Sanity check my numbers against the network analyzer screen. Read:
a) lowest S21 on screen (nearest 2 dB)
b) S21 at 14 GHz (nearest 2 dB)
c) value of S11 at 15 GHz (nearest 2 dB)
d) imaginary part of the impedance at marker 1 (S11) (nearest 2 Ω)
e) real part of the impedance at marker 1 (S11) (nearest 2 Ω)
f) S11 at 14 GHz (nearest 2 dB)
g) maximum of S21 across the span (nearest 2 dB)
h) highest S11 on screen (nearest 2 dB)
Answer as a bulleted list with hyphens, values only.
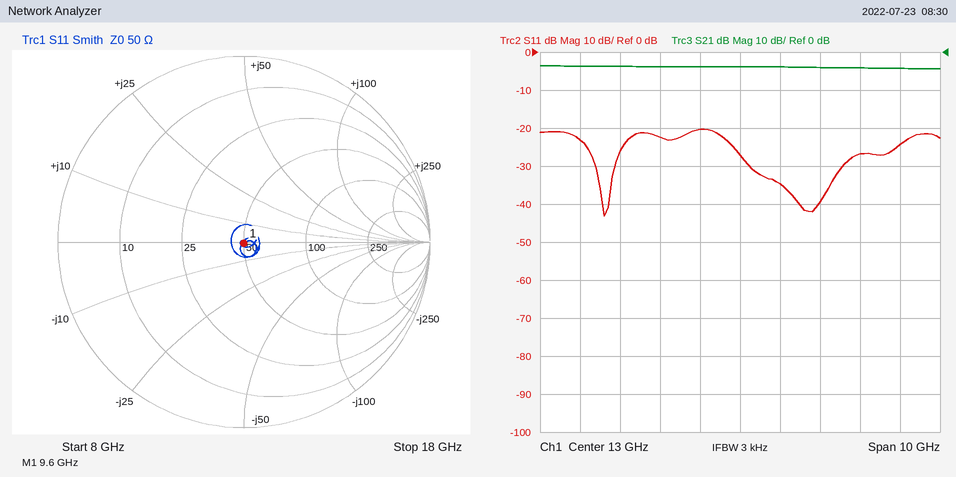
- -4 dB
- -4 dB
- -40 dB
- 0 Ω
- 50 Ω
- -34 dB
- -4 dB
- -20 dB
